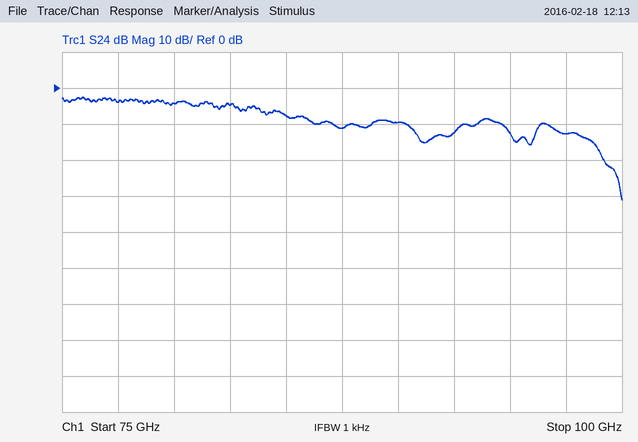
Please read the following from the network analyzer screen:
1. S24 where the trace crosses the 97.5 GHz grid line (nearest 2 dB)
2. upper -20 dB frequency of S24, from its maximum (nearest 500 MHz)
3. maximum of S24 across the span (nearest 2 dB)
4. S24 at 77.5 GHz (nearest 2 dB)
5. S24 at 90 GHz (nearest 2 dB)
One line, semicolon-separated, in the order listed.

-12 dB; 99.5 GHz; -2 dB; -4 dB; -10 dB
